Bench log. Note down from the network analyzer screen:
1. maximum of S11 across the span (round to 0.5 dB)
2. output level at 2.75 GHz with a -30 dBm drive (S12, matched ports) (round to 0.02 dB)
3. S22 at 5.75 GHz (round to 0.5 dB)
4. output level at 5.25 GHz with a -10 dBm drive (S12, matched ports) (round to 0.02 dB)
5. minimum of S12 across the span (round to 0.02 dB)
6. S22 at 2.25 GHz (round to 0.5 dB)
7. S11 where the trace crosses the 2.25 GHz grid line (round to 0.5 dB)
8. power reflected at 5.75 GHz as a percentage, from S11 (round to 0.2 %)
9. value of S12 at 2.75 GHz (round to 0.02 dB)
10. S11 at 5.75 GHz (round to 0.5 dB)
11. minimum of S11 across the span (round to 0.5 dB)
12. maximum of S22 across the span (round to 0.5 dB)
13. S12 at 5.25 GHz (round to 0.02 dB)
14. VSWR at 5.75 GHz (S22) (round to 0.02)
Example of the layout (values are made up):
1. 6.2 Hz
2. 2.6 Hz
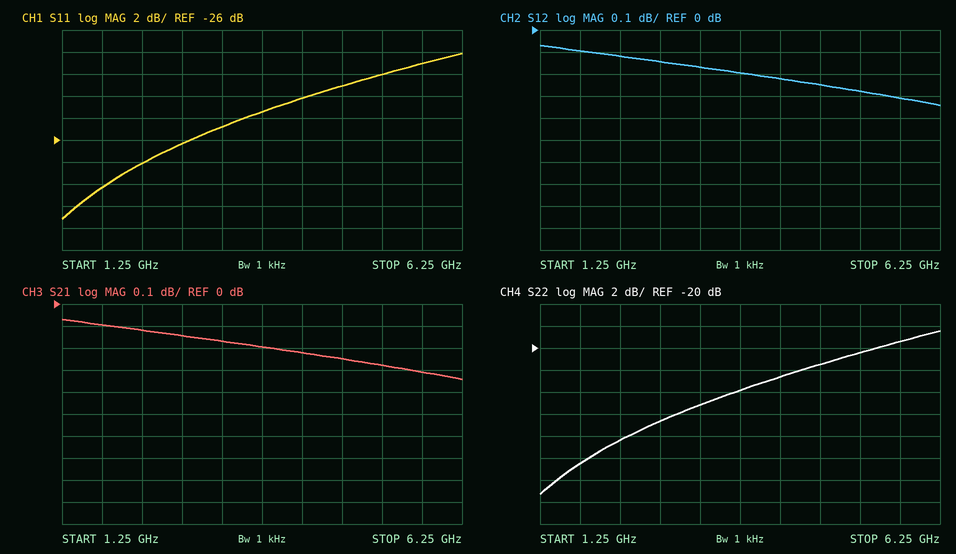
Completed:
1. -18.0 dB
2. -30.14 dBm
3. -19.5 dB
4. -10.28 dBm
5. -0.34 dB
6. -28.5 dB
7. -28.0 dB
8. 1.2 %
9. -0.14 dB
10. -19.0 dB
11. -33.0 dB
12. -18.5 dB
13. -0.28 dB
14. 1.24
